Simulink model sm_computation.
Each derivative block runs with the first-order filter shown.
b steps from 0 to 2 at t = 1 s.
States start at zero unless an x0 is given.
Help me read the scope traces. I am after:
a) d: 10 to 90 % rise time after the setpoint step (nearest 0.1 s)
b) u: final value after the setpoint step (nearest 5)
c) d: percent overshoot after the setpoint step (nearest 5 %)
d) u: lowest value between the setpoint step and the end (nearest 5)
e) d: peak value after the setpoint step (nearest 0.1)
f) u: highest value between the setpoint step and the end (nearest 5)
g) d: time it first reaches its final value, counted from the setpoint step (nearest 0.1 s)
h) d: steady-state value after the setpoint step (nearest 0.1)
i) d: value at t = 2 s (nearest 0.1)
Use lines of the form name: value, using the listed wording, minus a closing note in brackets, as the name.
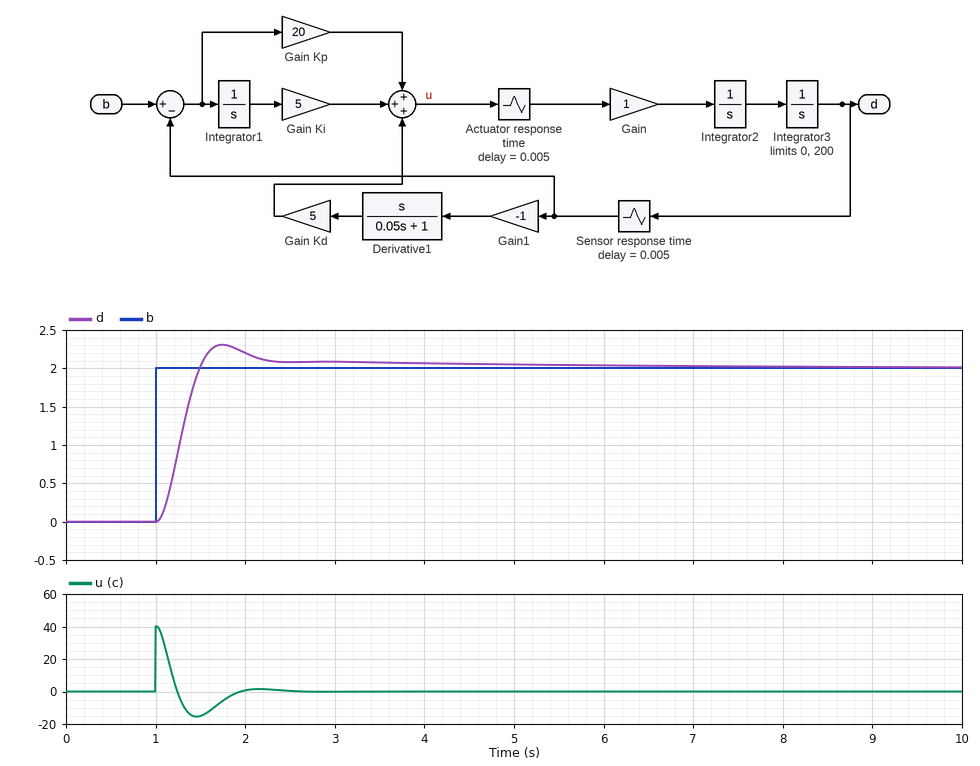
d: 10 to 90 % rise time after the setpoint step: 0.3 s
u: final value after the setpoint step: 0
d: percent overshoot after the setpoint step: 15 %
u: lowest value between the setpoint step and the end: -15
d: peak value after the setpoint step: 2.3
u: highest value between the setpoint step and the end: 40
d: time it first reaches its final value, counted from the setpoint step: 0.5 s
d: steady-state value after the setpoint step: 2.0
d: value at t = 2 s: 2.2
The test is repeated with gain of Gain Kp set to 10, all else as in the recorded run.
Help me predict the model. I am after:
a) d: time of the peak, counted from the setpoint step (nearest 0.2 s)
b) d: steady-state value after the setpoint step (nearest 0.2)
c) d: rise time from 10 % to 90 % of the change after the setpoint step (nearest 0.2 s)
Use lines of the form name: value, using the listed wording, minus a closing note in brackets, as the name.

d: time of the peak, counted from the setpoint step: 1.6 s
d: steady-state value after the setpoint step: 2.0
d: rise time from 10 % to 90 % of the change after the setpoint step: 0.6 s
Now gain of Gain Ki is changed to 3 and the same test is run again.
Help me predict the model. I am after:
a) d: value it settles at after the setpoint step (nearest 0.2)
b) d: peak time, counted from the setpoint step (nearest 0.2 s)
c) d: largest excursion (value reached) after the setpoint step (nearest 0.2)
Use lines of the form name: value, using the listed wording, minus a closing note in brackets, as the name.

d: value it settles at after the setpoint step: 2.0
d: peak time, counted from the setpoint step: 0.8 s
d: largest excursion (value reached) after the setpoint step: 2.2
